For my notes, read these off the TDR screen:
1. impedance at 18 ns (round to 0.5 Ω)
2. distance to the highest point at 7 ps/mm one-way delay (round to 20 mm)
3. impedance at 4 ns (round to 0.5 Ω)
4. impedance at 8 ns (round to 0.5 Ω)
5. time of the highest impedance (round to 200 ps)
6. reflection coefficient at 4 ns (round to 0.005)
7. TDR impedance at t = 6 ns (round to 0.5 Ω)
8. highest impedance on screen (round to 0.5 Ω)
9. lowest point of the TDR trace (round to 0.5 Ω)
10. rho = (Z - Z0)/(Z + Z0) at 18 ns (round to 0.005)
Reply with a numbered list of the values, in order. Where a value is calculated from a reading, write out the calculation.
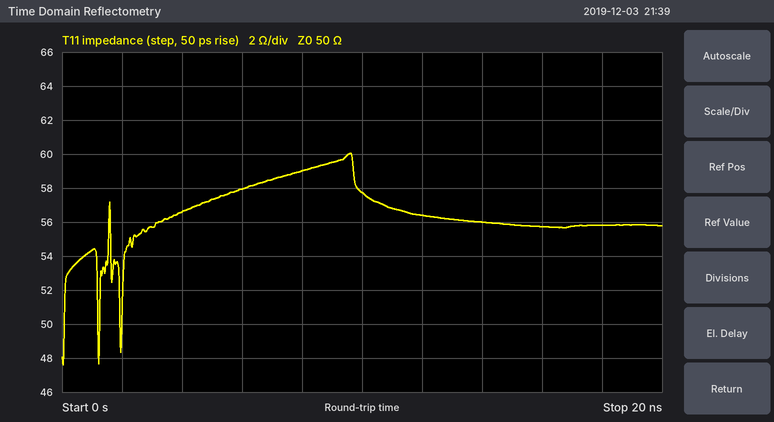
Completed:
1. 56.0 Ω
2. 9.6 ns / 2 / 7 ps/mm ≈ 686 mm, so 680 mm to the nearest 20 mm
3. 56.5 Ω
4. 59.0 Ω
5. 9.6 ns
6. (56.5 − 50)/(56.5 + 50) ≈ +0.0610, so +0.060 to the nearest 0.005
7. 58.0 Ω
8. 60.0 Ω
9. 47.5 Ω
10. (56 − 50)/(56 + 50) ≈ +0.0566, so +0.055 to the nearest 0.005
